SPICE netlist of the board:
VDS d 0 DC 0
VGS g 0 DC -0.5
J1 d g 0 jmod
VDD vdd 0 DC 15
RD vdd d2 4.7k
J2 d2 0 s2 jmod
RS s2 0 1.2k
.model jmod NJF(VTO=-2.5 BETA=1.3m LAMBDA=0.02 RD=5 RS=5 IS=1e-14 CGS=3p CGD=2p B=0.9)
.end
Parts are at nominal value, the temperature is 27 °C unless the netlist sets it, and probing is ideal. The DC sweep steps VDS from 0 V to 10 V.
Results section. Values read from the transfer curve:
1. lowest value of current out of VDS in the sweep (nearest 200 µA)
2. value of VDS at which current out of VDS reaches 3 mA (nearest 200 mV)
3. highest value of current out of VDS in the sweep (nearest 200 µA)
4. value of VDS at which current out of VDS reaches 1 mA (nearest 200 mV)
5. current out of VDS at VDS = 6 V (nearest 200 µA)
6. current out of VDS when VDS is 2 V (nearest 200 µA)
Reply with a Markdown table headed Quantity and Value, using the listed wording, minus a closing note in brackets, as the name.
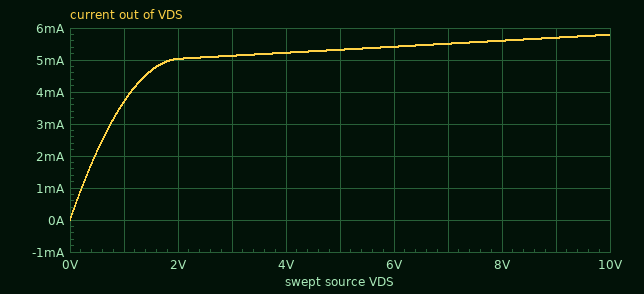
| Quantity | Value |
|---|---|
| lowest value of current out of VDS in the sweep | 0 A |
| value of VDS at which current out of VDS reaches 3 mA | 800 mV |
| highest value of current out of VDS in the sweep | 5.8 mA |
| value of VDS at which current out of VDS reaches 1 mA | 200 mV |
| current out of VDS at VDS = 6 V | 5.4 mA |
| current out of VDS when VDS is 2 V | 5.0 mA |
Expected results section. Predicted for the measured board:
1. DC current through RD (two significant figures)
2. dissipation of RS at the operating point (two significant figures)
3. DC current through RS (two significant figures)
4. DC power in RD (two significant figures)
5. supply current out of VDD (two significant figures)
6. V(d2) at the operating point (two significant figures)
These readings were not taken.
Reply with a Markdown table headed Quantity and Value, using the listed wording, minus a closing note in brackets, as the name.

| Quantity | Value |
|---|---|
| DC current through RD | 1.3 mA |
| dissipation of RS at the operating point | 2.0 mW |
| DC current through RS | 1.3 mA |
| DC power in RD | 7.7 mW |
| supply current out of VDD | 1.3 mA |
| V(d2) at the operating point | 9.0 V |
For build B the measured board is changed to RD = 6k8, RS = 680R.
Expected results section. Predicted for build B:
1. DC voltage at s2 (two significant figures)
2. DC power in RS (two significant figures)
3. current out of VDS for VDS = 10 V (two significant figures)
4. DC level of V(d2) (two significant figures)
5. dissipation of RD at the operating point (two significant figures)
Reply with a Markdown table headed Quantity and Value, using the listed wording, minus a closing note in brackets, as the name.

| Quantity | Value |
|---|---|
| DC voltage at s2 | 1.3 V |
| DC power in RS | 2.3 mW |
| current out of VDS for VDS = 10 V | 5.8 mA |
| DC level of V(d2) | 2.4 V |
| dissipation of RD at the operating point | 23 mW |
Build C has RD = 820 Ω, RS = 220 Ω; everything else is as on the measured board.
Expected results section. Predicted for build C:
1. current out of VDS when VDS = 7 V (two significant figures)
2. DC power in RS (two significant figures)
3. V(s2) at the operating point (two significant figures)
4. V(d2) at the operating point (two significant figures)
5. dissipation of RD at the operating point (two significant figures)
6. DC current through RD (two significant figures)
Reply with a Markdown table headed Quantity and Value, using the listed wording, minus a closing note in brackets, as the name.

| Quantity | Value |
|---|---|
| current out of VDS when VDS = 7 V | 5.5 mA |
| DC power in RS | 3.4 mW |
| V(s2) at the operating point | 860 mV |
| V(d2) at the operating point | 12 V |
| dissipation of RD at the operating point | 13 mW |
| DC current through RD | 3.9 mA |
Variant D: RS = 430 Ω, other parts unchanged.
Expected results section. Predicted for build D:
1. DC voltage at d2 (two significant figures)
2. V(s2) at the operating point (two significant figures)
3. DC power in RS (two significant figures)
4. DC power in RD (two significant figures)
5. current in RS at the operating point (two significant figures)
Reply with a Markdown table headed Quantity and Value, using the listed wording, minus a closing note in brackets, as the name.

| Quantity | Value |
|---|---|
| DC voltage at d2 | 3.2 V |
| V(s2) at the operating point | 1.1 V |
| DC power in RS | 2.7 mW |
| DC power in RD | 30 mW |
| current in RS at the operating point | 2.5 mA |
